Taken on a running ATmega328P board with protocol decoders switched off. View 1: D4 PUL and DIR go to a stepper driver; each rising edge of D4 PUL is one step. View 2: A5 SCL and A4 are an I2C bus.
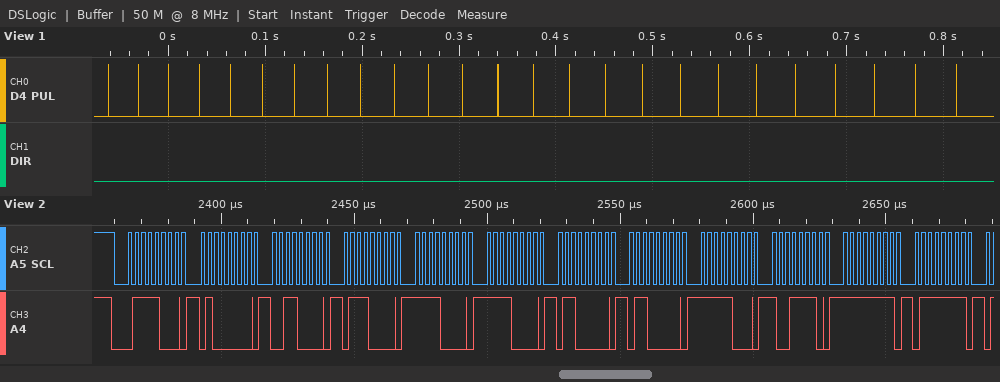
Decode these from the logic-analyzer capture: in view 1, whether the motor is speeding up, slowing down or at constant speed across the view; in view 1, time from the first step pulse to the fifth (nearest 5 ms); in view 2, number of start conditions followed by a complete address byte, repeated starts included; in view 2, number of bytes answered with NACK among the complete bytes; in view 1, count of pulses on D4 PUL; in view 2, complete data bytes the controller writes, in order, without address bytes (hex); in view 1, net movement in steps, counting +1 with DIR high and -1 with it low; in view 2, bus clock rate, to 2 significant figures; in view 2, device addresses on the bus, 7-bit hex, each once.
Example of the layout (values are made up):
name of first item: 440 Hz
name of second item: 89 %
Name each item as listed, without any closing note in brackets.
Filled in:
in view 1, whether the motor is speeding up, slowing down or at constant speed across the view: slowing down
in view 1, time from the first step pulse to the fifth: 125 ms
in view 2, number of start conditions followed by a complete address byte, repeated starts included: 1
in view 2, number of bytes answered with NACK among the complete bytes: 0
in view 1, count of pulses on D4 PUL: 25
in view 2, complete data bytes the controller writes, in order, without address bytes: 40 30 70 F0 F0 60 60 F8 9E FF 7F
in view 1, net movement in steps, counting +1 with DIR high and -1 with it low: -25
in view 2, bus clock rate, to 2 significant figures: 400 kHz
in view 2, device addresses on the bus, 7-bit hex, each once: 0x3C
